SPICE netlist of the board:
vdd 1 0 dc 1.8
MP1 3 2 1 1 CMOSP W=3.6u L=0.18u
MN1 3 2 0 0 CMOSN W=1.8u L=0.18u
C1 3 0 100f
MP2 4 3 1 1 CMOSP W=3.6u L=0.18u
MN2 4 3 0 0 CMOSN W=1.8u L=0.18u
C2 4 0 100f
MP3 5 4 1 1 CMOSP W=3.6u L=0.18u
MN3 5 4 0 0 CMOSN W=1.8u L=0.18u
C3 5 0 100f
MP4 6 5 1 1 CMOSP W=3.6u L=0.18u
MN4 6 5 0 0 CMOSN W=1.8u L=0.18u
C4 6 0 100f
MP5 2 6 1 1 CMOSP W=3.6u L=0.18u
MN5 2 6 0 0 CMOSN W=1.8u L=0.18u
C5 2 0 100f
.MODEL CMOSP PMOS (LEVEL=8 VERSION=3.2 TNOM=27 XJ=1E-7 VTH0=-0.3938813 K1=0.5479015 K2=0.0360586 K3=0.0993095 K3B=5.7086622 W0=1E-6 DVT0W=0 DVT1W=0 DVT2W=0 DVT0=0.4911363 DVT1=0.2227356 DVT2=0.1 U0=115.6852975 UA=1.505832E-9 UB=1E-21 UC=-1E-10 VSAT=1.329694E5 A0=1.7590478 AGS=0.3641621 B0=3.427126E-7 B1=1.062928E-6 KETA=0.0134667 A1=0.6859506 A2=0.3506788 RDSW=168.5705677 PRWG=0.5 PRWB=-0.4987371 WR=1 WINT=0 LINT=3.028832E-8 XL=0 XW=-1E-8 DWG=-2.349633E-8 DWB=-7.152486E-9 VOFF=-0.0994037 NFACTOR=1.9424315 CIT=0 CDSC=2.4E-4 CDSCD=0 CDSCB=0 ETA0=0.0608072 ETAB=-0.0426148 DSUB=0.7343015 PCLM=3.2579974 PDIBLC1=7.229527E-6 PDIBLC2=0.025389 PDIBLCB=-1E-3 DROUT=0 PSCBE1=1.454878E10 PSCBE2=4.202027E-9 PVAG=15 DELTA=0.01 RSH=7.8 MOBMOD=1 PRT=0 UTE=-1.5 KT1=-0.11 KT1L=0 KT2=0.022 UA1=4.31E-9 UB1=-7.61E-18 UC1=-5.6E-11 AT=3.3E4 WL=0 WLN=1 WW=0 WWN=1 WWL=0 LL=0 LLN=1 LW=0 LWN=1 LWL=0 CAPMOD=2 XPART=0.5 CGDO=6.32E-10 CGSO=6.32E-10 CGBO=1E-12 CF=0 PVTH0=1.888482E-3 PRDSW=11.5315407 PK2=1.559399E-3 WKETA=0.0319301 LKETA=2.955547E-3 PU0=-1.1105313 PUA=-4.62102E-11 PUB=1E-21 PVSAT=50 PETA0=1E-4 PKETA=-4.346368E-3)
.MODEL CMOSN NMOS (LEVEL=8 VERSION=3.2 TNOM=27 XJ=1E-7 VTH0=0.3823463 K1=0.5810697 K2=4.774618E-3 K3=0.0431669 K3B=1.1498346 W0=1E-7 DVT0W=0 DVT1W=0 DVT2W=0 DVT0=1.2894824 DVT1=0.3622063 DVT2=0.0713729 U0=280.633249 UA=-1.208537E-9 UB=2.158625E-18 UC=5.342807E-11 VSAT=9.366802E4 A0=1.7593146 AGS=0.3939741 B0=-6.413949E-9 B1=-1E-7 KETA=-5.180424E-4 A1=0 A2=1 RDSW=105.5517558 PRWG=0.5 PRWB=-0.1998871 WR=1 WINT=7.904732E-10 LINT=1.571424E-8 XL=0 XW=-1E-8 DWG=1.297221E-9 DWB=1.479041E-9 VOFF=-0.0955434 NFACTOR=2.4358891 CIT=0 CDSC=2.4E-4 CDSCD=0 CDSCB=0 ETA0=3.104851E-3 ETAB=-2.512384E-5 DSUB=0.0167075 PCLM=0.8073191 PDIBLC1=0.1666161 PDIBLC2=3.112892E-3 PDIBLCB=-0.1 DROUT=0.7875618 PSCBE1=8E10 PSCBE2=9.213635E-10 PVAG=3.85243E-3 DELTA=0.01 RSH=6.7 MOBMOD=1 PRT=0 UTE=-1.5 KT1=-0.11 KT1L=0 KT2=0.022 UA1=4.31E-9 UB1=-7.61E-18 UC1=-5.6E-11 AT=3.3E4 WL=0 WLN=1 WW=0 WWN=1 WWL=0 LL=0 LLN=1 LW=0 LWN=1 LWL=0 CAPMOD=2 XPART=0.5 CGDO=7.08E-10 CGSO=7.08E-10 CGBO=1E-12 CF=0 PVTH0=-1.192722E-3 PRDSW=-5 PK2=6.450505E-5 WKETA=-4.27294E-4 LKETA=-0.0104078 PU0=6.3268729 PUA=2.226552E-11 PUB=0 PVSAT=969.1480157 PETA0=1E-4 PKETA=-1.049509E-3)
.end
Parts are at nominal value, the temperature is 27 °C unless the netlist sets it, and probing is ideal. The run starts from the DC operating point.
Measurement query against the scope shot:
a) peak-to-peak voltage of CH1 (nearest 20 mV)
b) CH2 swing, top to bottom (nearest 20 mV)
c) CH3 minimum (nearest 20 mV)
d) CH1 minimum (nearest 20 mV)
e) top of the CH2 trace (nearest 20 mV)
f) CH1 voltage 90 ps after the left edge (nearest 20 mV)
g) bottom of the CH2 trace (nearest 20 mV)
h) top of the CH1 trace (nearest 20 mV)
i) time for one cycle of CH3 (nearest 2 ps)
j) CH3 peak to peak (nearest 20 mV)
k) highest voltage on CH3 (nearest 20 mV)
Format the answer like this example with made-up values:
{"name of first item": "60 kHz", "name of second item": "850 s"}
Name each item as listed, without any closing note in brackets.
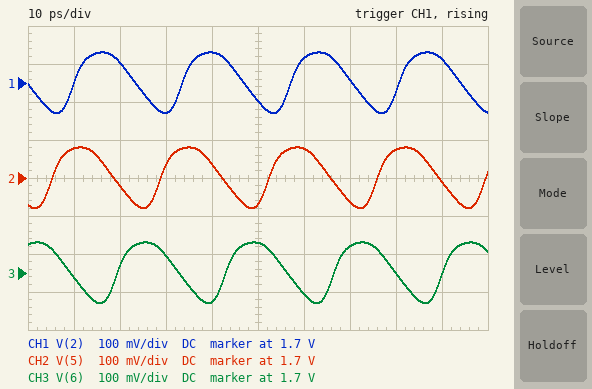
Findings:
{"peak-to-peak voltage of CH1": "160 mV", "CH2 swing, top to bottom": "160 mV", "CH3 minimum": "1.62 V", "CH1 minimum": "1.62 V", "top of the CH2 trace": "1.78 V", "CH1 voltage 90 ps after the left edge": "1.76 V", "bottom of the CH2 trace": "1.62 V", "top of the CH1 trace": "1.78 V", "time for one cycle of CH3": "24 ps", "CH3 peak to peak": "160 mV", "highest voltage on CH3": "1.78 V"}
